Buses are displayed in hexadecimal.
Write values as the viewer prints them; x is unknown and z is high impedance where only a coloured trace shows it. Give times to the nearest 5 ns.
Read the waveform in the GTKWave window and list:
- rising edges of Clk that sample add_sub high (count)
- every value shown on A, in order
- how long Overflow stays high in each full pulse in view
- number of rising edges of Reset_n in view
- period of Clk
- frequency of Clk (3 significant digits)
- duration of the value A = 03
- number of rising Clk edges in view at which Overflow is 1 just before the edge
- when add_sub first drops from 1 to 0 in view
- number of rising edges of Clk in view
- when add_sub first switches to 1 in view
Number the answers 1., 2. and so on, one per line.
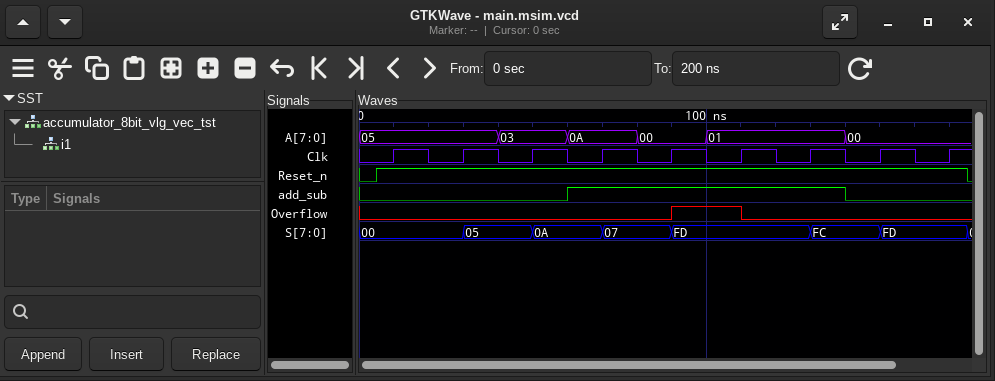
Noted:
1. 4
2. 05, 03, 0A, 00, 01, 00
3. 20 ns
4. 1
5. 20 ns
6. 50.0 MHz
7. 20 ns
8. 1
9. 140 ns
10. 9
11. 60 ns
